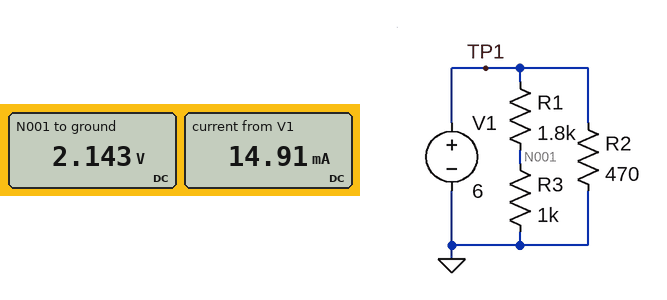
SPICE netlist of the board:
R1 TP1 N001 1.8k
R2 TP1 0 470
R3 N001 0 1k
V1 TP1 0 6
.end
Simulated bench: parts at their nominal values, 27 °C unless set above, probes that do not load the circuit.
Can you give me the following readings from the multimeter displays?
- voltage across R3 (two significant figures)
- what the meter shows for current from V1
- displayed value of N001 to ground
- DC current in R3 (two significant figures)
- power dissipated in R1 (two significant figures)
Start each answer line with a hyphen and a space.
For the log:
- 2.1 V
- 14.91 mA
- 2.143 V
- 2.1 mA
- 8.3 mW
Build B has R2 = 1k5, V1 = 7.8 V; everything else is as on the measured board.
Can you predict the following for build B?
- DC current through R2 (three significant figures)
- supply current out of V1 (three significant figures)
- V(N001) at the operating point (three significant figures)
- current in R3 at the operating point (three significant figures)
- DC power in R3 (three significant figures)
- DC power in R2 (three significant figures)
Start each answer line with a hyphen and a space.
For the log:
- 5.20 mA
- 7.99 mA
- 2.79 V
- 2.79 mA
- 7.76 mW
- 40.6 mW
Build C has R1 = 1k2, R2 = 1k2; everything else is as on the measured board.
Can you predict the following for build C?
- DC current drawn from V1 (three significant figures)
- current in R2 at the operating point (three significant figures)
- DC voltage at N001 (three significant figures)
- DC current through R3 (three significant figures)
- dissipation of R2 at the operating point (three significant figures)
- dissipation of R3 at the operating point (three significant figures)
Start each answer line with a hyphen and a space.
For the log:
- 7.73 mA
- 5.00 mA
- 2.73 V
- 2.73 mA
- 30.0 mW
- 7.44 mW
